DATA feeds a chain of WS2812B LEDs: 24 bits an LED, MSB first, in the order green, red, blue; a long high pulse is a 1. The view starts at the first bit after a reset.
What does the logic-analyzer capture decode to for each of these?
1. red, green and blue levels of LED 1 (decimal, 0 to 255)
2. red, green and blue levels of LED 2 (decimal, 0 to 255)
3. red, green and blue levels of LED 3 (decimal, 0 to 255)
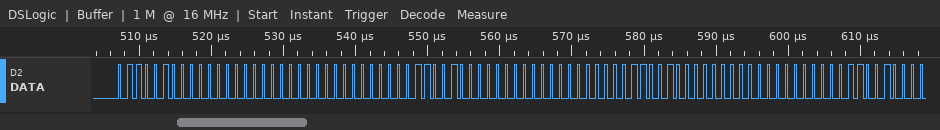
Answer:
0, 100, 0
100, 0, 0
100, 0, 0
